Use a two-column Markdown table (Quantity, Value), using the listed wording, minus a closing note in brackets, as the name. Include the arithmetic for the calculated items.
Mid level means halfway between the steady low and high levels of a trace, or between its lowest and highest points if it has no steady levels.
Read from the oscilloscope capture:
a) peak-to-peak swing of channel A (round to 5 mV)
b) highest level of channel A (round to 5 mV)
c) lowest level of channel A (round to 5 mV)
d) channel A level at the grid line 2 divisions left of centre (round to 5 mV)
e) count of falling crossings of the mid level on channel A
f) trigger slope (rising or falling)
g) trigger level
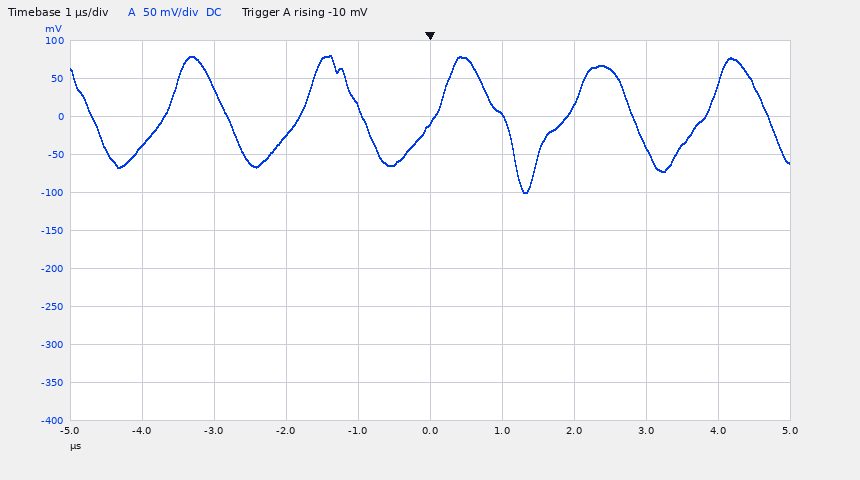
| Quantity | Value |
|---|---|
| peak-to-peak swing of channel A | 80 mV − (-100 mV) = 180 mV |
| highest level of channel A | 80 mV |
| lowest level of channel A | -100 mV |
| channel A level at the grid line 2 divisions left of centre | -25 mV |
| count of falling crossings of the mid level on channel A | 6 |
| trigger slope | rising |
| trigger level | -10 mV |
